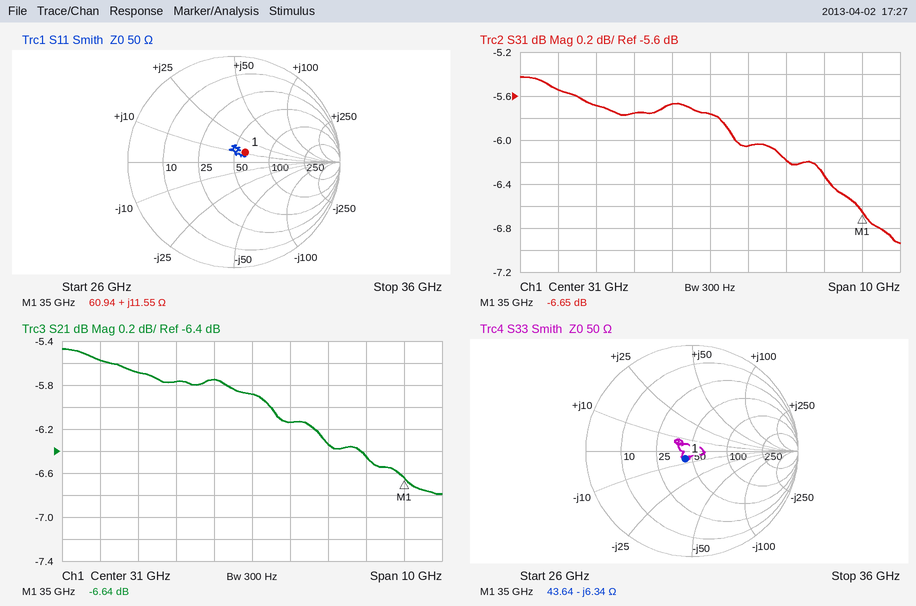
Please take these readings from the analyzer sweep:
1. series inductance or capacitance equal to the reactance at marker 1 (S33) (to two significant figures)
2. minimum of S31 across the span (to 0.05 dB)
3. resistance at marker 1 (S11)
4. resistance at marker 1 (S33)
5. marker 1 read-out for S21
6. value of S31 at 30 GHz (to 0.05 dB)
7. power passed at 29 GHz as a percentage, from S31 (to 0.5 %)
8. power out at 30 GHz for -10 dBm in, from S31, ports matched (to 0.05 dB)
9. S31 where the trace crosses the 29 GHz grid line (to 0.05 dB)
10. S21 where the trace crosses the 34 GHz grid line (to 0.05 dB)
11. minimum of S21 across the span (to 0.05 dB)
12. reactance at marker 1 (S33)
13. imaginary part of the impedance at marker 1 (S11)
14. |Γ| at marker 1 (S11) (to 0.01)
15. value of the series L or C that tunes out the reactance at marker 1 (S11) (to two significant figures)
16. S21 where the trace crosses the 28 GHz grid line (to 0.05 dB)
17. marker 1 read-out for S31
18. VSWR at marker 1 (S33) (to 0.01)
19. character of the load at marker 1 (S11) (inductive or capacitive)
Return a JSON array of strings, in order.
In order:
["720 fF", "-6.95 dB", "60.94 Ω", "43.64 Ω", "-6.64 dB", "-5.65 dB", "26.5 %", "-15.65 dBm", "-5.75 dB", "-6.45 dB", "-6.80 dB", "-6.34 Ω", "+11.55 Ω", "0.14", "390 fF", "-5.70 dB", "-6.65 dB", "1.21", "inductive"]
